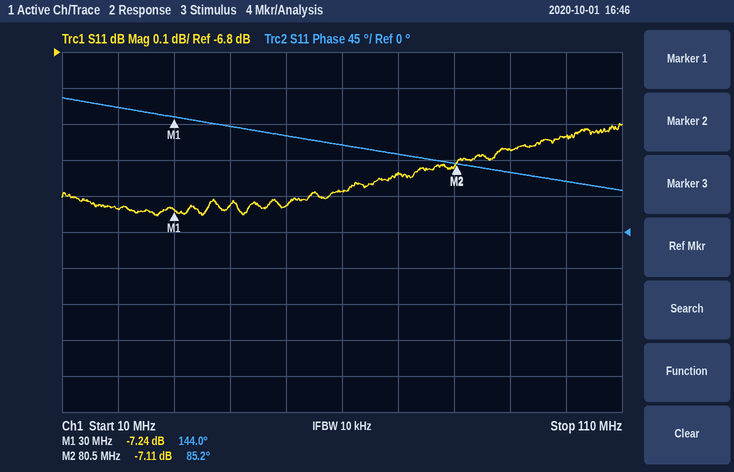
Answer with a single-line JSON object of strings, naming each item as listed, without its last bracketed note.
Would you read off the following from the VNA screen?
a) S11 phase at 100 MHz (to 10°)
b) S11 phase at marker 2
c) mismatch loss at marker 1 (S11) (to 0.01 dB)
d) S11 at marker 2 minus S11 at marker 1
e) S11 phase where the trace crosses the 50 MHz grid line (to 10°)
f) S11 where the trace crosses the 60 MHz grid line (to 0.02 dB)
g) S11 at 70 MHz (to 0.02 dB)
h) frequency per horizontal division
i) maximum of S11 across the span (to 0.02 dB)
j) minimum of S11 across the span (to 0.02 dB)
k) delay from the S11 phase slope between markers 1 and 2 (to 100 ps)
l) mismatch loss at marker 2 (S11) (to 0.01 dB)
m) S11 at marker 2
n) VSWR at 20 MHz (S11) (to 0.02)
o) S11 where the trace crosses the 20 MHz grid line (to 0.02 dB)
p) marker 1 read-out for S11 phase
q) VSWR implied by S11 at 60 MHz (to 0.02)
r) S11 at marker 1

{"S11 phase at 100 MHz": "60°", "S11 phase at marker 2": "85.2°", "mismatch loss at marker 1 (S11)": "0.91 dB", "S11 at marker 2 minus S11 at marker 1": "0.13 dB", "S11 phase where the trace crosses the 50 MHz grid line": "120°", "S11 where the trace crosses the 60 MHz grid line": "-7.18 dB", "S11 at 70 MHz": "-7.14 dB", "frequency per horizontal division": "10 MHz", "maximum of S11 across the span": "-7.00 dB", "minimum of S11 across the span": "-7.26 dB", "delay from the S11 phase slope between markers 1 and 2": "3.2 ns", "mismatch loss at marker 2 (S11)": "0.94 dB", "S11 at marker 2": "-7.11 dB", "VSWR at 20 MHz (S11)": "2.54", "S11 where the trace crosses the 20 MHz grid line": "-7.24 dB", "marker 1 read-out for S11 phase": "144.0°", "VSWR implied by S11 at 60 MHz": "2.56", "S11 at marker 1": "-7.24 dB"}
